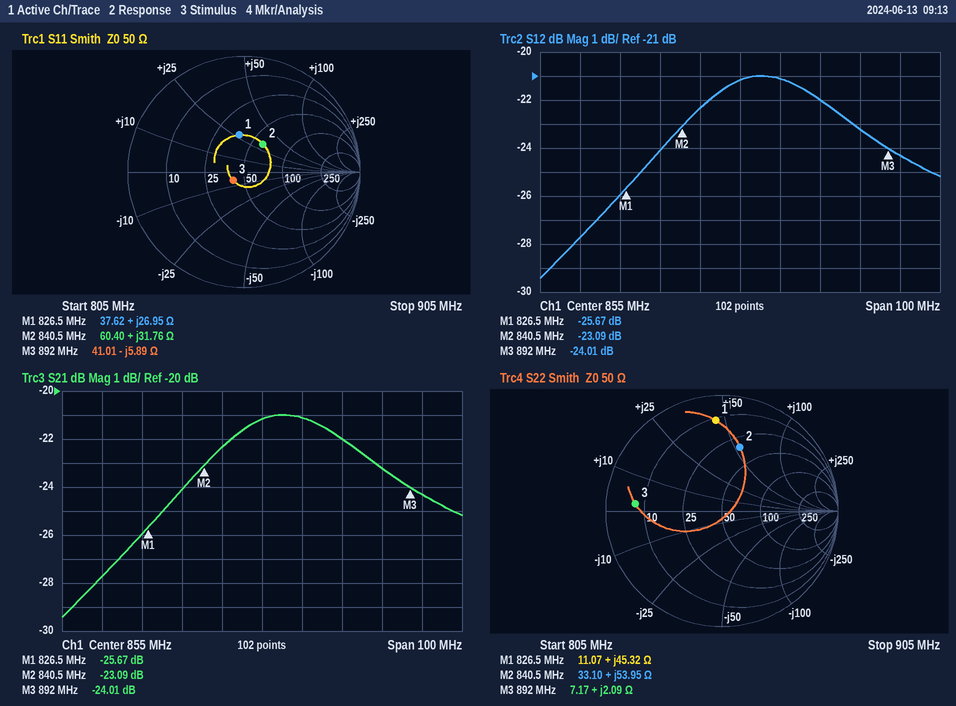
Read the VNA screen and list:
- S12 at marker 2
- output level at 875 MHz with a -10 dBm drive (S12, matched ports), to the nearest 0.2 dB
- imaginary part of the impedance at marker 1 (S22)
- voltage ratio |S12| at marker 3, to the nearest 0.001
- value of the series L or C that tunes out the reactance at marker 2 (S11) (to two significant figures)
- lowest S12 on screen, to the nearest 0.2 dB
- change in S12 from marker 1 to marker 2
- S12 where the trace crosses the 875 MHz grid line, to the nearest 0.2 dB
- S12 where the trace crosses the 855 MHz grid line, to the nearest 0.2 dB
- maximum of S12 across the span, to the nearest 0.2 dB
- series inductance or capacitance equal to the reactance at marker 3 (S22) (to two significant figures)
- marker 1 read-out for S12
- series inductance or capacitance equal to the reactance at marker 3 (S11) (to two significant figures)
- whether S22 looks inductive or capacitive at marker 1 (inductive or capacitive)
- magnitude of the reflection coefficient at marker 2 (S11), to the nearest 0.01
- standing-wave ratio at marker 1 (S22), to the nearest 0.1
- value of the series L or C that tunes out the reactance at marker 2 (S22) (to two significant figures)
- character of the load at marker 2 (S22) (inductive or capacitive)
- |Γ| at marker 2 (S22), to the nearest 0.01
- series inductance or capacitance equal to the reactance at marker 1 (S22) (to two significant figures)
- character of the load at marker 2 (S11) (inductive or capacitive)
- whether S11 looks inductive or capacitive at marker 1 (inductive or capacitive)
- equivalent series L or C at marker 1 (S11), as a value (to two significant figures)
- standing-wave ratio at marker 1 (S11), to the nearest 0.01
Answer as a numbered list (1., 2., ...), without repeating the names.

1. -23.09 dB
2. -32.0 dBm
3. +45.32 Ω
4. 0.063
5. 6.0 pF
6. -29.4 dB
7. 2.58 dB
8. -22.0 dB
9. -21.2 dB
10. -21.0 dB
11. 370 pH
12. -25.67 dB
13. 30 pF
14. inductive
15. 0.29
16. 8.3
17. 3.5 pF
18. inductive
19. 0.57
20. 8.7 nH
21. inductive
22. inductive
23. 5.2 nH
24. 1.96
